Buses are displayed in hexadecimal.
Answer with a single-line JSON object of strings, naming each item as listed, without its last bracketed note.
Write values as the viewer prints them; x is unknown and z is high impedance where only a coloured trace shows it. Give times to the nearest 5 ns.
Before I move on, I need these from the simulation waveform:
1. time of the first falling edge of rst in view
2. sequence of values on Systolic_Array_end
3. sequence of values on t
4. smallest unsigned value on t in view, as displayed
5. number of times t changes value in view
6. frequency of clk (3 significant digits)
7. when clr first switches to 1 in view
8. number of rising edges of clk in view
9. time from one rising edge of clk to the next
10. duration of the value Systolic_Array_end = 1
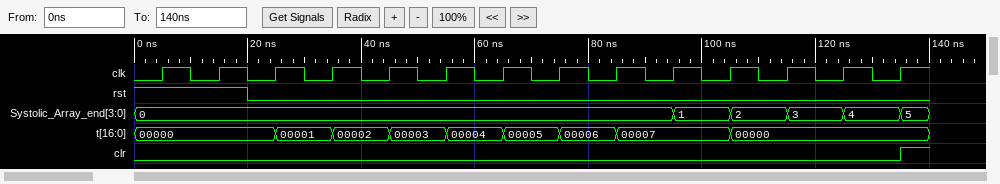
{"time of the first falling edge of rst in view": "20 ns", "sequence of values on Systolic_Array_end": "0, 1, 2, 3, 4, 5", "sequence of values on t": "00000, 00001, 00002, 00003, 00004, 00005, 00006, 00007, 00000", "smallest unsigned value on t in view, as displayed": "00000", "number of times t changes value in view": "8", "frequency of clk": "100 MHz", "when clr first switches to 1 in view": "135 ns", "number of rising edges of clk in view": "14", "time from one rising edge of clk to the next": "10 ns", "duration of the value Systolic_Array_end = 1": "10 ns"}
